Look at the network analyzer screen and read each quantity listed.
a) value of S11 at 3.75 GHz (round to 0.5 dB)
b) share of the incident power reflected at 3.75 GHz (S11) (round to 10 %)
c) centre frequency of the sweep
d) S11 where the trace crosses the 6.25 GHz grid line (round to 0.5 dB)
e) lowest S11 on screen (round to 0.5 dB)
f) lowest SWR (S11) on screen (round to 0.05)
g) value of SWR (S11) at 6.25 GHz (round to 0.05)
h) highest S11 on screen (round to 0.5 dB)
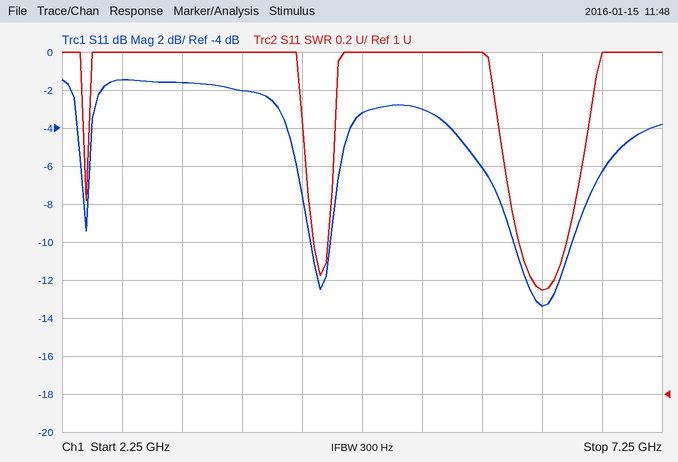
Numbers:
-2.0 dB
60 %
4.75 GHz
-13.5 dB
-13.5 dB
1.55
1.55
-1.5 dB
